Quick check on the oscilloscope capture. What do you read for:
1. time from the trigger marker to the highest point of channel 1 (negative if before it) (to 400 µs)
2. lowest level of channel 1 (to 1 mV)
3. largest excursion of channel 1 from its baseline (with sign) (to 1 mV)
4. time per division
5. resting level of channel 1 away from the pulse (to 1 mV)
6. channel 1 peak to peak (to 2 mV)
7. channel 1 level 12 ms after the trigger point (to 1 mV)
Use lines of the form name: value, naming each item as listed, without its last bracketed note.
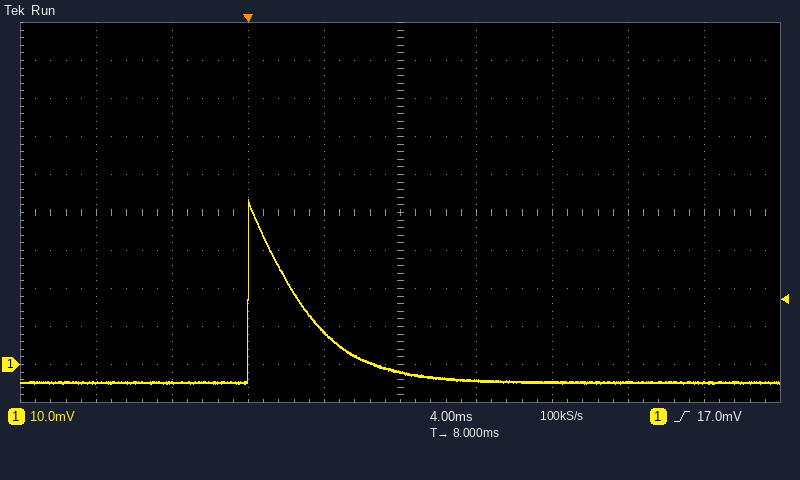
time from the trigger marker to the highest point of channel 1 (negative if before it): 0.0 ms
lowest level of channel 1: -5 mV
largest excursion of channel 1 from its baseline (with sign): +48 mV
time per division: 4 ms
resting level of channel 1 away from the pulse: -5 mV
channel 1 peak to peak: 48 mV
channel 1 level 12 ms after the trigger point: -4 mV
